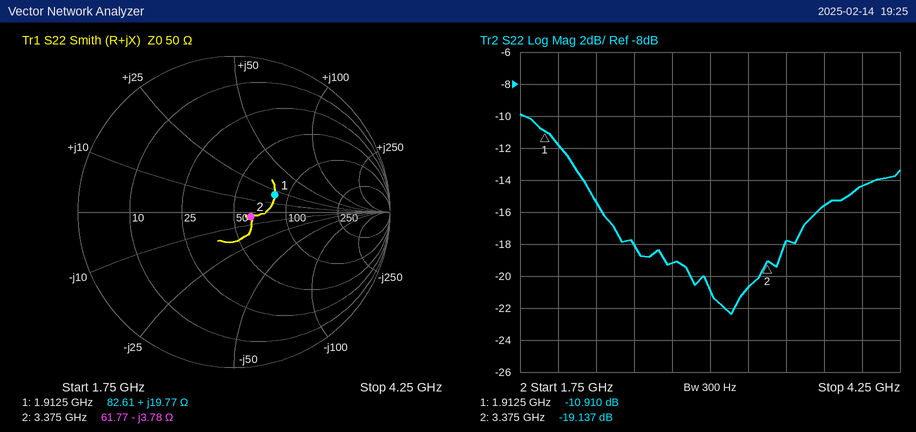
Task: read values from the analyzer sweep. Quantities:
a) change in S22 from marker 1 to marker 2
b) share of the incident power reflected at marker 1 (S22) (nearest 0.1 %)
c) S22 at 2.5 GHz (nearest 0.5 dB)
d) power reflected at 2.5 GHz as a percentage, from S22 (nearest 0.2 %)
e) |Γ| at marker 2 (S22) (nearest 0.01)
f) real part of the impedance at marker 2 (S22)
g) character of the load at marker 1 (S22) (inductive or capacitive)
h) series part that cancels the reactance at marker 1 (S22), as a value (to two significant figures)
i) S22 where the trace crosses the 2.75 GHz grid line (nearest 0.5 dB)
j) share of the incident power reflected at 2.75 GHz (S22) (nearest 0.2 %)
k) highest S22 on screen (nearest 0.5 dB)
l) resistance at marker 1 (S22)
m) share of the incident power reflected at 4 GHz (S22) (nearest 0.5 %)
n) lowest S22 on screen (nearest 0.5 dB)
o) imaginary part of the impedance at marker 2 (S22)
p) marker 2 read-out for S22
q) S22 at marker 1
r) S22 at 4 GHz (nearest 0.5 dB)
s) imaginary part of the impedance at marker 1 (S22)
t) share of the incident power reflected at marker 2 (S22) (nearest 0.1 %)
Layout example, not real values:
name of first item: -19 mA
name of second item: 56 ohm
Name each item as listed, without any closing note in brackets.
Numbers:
change in S22 from marker 1 to marker 2: -8.227 dB
share of the incident power reflected at marker 1 (S22): 8.1 %
S22 at 2.5 GHz: -18.0 dB
power reflected at 2.5 GHz as a percentage, from S22: 1.6 %
|Γ| at marker 2 (S22): 0.11
real part of the impedance at marker 2: 61.77 Ω
character of the load at marker 1 (S22): inductive
series part that cancels the reactance at marker 1 (S22), as a value: 4.2 pF
S22 where the trace crosses the 2.75 GHz grid line: -19.0 dB
share of the incident power reflected at 2.75 GHz (S22): 1.2 %
highest S22 on screen: -10.0 dB
resistance at marker 1: 82.61 Ω
share of the incident power reflected at 4 GHz (S22): 3.5 %
lowest S22 on screen: -22.5 dB
imaginary part of the impedance at marker 2: -3.78 Ω
marker 2 read-out for S22: -19.137 dB
S22 at marker 1: -10.910 dB
S22 at 4 GHz: -14.5 dB
imaginary part of the impedance at marker 1: +19.77 Ω
share of the incident power reflected at marker 2 (S22): 1.2 %
